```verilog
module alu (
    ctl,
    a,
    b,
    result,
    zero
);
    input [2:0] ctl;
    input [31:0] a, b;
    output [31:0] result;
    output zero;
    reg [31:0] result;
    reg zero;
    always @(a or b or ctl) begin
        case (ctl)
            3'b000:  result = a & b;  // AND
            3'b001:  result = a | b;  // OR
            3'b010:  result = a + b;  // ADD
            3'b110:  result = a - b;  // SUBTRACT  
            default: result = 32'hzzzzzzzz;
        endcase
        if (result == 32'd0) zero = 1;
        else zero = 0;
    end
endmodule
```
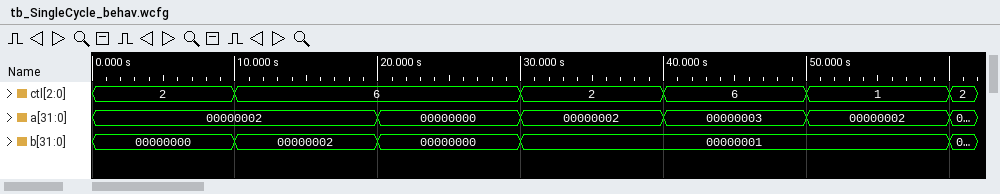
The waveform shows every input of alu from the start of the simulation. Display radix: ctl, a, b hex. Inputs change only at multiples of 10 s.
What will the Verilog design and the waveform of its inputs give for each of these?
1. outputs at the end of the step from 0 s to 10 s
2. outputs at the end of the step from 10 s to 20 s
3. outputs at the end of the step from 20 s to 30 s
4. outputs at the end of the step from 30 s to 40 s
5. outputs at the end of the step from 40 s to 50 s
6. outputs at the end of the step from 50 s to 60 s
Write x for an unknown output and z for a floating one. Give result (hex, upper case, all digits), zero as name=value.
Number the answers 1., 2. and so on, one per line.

1. result=00000002, zero=0
2. result=00000000, zero=1
3. result=00000000, zero=1
4. result=00000003, zero=0
5. result=00000002, zero=0
6. result=00000003, zero=0
